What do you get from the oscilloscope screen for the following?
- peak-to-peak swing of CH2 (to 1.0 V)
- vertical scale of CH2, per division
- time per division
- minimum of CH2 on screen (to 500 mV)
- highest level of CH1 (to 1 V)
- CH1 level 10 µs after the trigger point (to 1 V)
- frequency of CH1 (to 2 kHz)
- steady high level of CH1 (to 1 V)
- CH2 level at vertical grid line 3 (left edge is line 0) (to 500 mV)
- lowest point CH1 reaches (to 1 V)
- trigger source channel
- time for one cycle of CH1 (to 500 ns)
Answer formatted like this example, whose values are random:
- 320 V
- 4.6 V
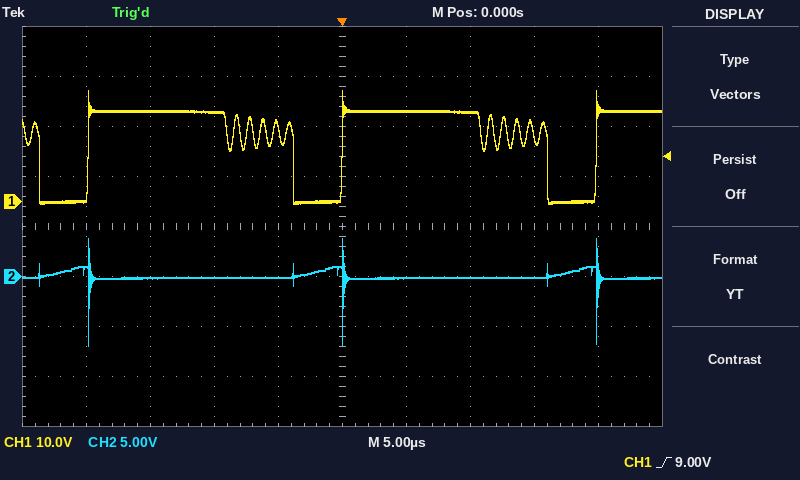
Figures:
- 11.0 V
- 5 V
- 5 µs
- -7.0 V
- 22 V
- 18 V
- 50 kHz
- 18 V
- 0.0 V
- 0 V
- CH1
- 20.0 µs
